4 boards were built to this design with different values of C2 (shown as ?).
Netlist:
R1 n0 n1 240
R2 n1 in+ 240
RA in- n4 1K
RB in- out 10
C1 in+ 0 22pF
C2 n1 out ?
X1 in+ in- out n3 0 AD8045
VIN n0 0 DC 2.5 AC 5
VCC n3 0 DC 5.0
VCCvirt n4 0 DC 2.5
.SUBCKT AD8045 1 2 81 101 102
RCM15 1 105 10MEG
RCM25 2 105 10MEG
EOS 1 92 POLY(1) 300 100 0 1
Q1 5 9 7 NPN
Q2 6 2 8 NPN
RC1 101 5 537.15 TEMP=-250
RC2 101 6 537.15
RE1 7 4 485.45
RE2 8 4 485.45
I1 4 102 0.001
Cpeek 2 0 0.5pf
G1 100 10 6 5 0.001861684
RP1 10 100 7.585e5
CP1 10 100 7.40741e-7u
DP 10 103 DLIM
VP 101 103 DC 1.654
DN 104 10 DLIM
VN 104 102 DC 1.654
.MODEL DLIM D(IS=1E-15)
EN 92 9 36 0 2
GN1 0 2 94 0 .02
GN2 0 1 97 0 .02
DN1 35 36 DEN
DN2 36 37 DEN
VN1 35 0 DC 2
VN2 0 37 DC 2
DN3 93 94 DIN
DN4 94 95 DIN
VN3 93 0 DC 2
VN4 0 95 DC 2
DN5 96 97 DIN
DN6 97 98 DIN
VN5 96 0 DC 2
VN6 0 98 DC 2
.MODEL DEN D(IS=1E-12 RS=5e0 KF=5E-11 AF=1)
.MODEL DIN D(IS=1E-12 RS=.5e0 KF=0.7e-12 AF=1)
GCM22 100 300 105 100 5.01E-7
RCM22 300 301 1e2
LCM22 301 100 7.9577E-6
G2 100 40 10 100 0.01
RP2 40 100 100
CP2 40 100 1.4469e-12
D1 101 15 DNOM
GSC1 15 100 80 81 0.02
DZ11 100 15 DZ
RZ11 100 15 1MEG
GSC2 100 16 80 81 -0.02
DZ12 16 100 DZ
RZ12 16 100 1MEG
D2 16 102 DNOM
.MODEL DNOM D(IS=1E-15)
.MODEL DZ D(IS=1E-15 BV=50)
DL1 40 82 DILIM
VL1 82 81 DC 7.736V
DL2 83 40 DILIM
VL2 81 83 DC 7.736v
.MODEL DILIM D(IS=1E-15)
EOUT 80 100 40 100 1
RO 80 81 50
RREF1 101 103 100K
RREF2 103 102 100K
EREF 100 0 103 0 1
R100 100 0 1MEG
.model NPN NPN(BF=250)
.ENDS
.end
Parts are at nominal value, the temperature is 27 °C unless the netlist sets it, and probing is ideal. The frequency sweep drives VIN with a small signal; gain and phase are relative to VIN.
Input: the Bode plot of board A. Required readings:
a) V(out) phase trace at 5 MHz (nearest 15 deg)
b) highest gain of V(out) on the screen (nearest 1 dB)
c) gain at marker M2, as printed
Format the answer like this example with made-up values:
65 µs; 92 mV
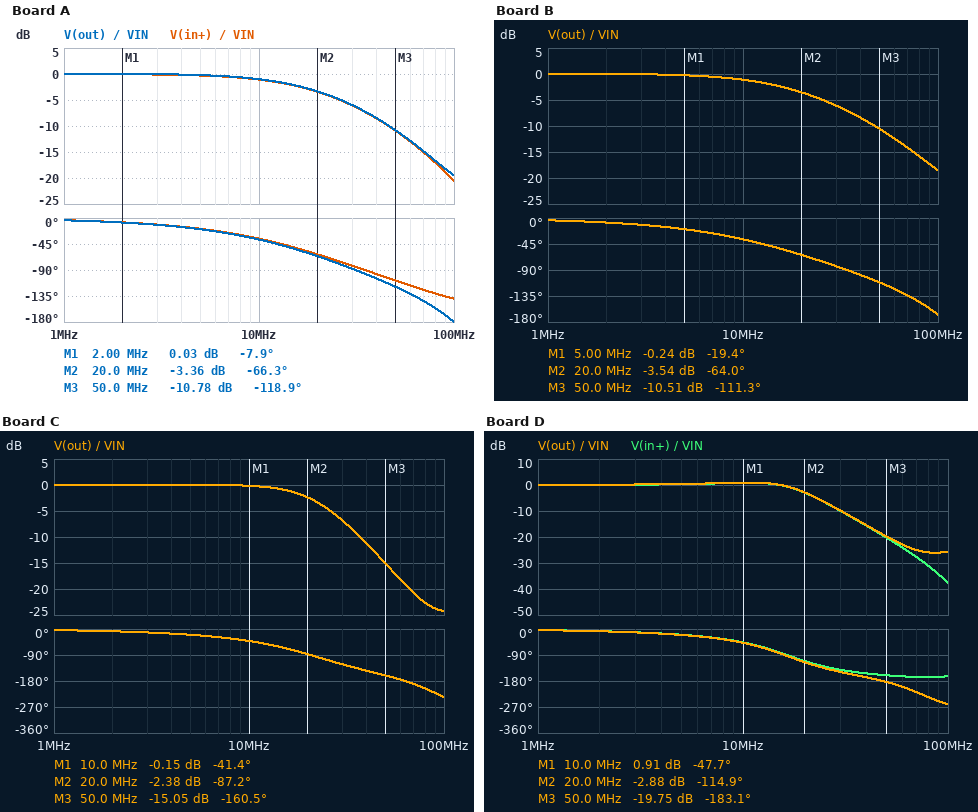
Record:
-15 deg; 0 dB; -3.36 dB
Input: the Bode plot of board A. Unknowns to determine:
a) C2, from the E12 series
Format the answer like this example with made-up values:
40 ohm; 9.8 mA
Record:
15 pF
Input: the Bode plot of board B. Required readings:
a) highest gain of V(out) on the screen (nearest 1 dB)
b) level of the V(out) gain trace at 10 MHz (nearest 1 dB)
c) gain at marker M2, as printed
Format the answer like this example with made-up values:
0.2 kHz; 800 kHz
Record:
0 dB; -1 dB; -3.54 dB
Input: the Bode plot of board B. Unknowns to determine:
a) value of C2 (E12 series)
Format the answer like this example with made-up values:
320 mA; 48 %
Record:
12 pF
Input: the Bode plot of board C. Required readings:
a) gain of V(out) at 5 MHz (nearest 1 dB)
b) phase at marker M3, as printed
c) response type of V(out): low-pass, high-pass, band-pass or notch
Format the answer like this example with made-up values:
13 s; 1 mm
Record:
0 dB; -160.5 deg; low-pass
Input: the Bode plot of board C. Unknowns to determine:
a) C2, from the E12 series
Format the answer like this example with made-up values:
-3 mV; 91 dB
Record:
39 pF
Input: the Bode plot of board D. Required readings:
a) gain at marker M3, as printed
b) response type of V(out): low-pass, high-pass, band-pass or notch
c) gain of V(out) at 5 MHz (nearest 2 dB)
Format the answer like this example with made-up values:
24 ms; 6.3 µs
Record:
-19.75 dB; low-pass; 0 dB
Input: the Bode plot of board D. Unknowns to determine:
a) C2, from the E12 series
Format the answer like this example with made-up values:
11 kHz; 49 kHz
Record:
68 pF
